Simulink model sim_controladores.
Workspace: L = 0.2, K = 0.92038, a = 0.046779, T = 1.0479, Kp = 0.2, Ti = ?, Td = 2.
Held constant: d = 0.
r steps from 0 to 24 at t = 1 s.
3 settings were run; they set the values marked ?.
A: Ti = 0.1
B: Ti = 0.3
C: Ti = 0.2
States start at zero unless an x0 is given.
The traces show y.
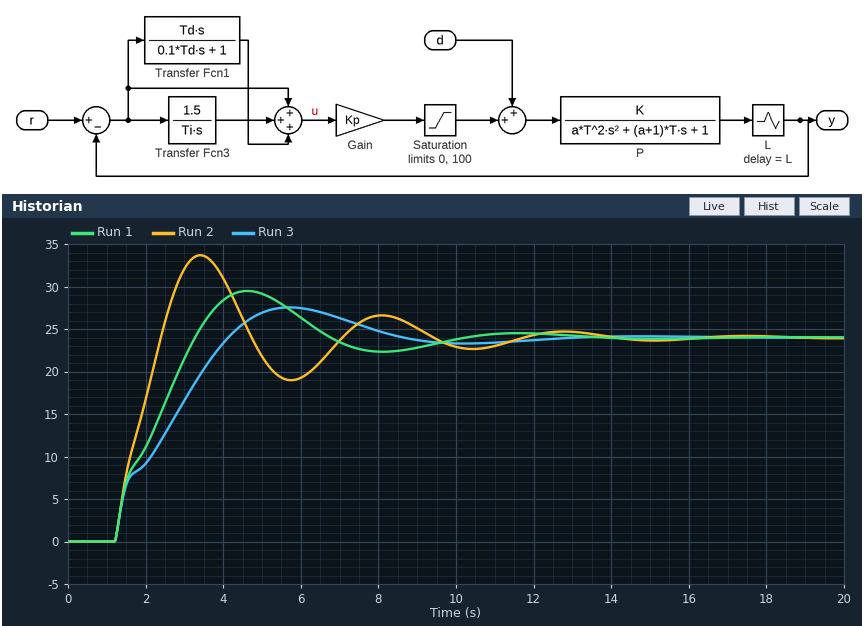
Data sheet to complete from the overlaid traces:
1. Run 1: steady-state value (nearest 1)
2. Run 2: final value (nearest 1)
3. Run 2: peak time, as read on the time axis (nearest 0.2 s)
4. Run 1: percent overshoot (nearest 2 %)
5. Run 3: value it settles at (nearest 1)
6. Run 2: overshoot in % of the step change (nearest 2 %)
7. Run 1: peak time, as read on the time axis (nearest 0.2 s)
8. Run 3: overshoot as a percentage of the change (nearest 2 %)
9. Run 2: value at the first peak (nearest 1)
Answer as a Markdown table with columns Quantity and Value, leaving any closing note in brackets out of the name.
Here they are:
| Quantity | Value |
|---|---|
| Run 1: steady-state value | 24 |
| Run 2: final value | 24 |
| Run 2: peak time, as read on the time axis | 3.4 s |
| Run 1: percent overshoot | 22 % |
| Run 3: value it settles at | 24 |
| Run 2: overshoot in % of the step change | 40 % |
| Run 1: peak time, as read on the time axis | 4.6 s |
| Run 3: overshoot as a percentage of the change | 14 % |
| Run 2: value at the first peak | 34 |
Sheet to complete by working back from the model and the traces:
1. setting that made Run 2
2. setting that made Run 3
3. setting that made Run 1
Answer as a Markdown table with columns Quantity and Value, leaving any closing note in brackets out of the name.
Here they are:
| Quantity | Value |
|---|---|
| setting that made Run 2 | A |
| setting that made Run 3 | B |
| setting that made Run 1 | C |
